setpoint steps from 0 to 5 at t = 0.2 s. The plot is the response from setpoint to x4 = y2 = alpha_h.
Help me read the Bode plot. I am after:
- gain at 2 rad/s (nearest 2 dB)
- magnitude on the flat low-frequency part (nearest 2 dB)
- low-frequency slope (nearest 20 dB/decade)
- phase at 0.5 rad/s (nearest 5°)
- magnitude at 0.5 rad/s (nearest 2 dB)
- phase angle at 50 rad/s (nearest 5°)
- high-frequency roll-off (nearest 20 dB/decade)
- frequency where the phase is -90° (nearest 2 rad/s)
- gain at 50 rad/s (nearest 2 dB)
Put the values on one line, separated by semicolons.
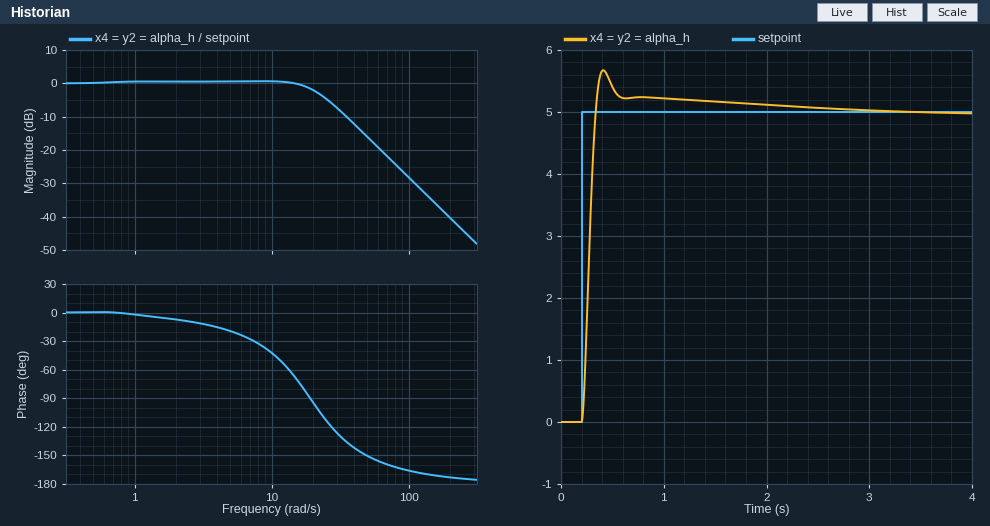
0 dB; 0 dB; 0 dB/decade; 0°; 0 dB; -150°; -40 dB/decade; 20 rad/s; -16 dB
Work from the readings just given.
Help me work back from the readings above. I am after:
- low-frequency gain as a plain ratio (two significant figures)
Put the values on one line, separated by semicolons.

1.0
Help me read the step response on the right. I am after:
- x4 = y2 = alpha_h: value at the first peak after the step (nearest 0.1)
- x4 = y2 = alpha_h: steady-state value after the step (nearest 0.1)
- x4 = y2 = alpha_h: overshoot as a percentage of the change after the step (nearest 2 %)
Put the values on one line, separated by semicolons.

5.7; 5.0; 14 %
